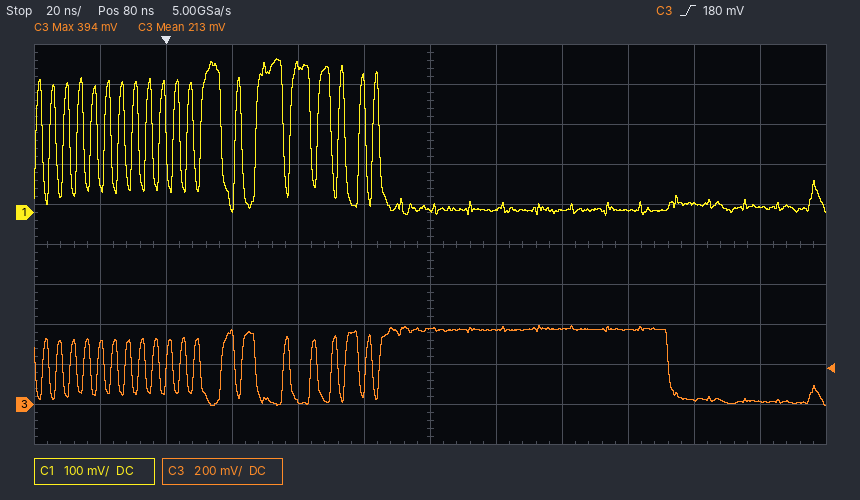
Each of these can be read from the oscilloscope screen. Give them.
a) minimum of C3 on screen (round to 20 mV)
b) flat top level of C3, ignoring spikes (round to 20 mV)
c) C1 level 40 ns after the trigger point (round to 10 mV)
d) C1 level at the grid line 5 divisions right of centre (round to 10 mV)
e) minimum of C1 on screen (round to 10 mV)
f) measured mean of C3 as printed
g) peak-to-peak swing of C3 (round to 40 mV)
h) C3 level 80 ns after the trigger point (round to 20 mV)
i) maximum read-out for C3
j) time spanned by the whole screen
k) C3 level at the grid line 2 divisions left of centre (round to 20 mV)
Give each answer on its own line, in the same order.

0 mV
380 mV
370 mV
10 mV
-10 mV
213 mV
400 mV
380 mV
394 mV
240 ns
20 mV
